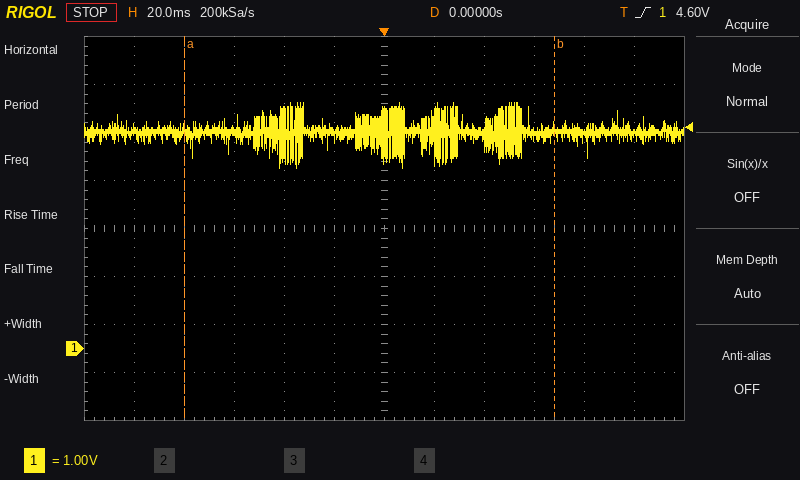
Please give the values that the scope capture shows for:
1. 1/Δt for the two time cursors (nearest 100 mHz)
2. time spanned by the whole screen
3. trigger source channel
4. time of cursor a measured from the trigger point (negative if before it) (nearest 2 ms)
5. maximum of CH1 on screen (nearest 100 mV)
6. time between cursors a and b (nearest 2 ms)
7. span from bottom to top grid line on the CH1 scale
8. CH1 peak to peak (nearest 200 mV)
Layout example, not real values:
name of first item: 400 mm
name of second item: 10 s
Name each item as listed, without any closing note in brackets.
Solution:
1/Δt for the two time cursors: 6.8 Hz
time spanned by the whole screen: 240 ms
trigger source channel: CH1
time of cursor a measured from the trigger point (negative if before it): -80 ms
maximum of CH1 on screen: 5.1 V
time between cursors a and b: 148 ms
span from bottom to top grid line on the CH1 scale: 8 V
CH1 peak to peak: 1.4 V
